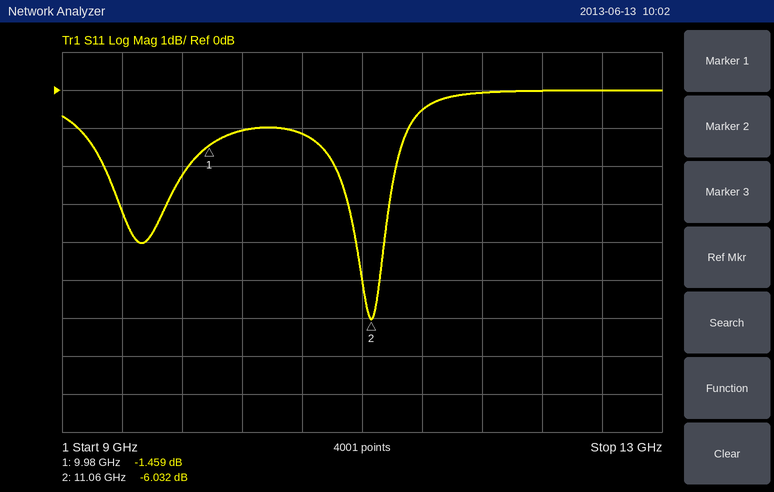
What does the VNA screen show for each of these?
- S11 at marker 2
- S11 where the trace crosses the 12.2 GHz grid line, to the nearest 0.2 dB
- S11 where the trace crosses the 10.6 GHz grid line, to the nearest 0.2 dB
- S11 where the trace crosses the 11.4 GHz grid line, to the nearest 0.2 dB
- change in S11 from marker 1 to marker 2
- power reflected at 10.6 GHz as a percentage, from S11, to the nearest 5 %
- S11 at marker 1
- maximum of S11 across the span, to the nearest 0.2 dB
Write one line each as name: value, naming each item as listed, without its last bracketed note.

S11 at marker 2: -6.032 dB
S11 where the trace crosses the 12.2 GHz grid line, to the nearest 0.2 dB: 0.0 dB
S11 where the trace crosses the 10.6 GHz grid line, to the nearest 0.2 dB: -1.2 dB
S11 where the trace crosses the 11.4 GHz grid line, to the nearest 0.2 dB: -0.6 dB
change in S11 from marker 1 to marker 2: -4.573 dB
power reflected at 10.6 GHz as a percentage, from S11, to the nearest 5 %: 75 %
S11 at marker 1: -1.459 dB
maximum of S11 across the span, to the nearest 0.2 dB: 0.0 dB
